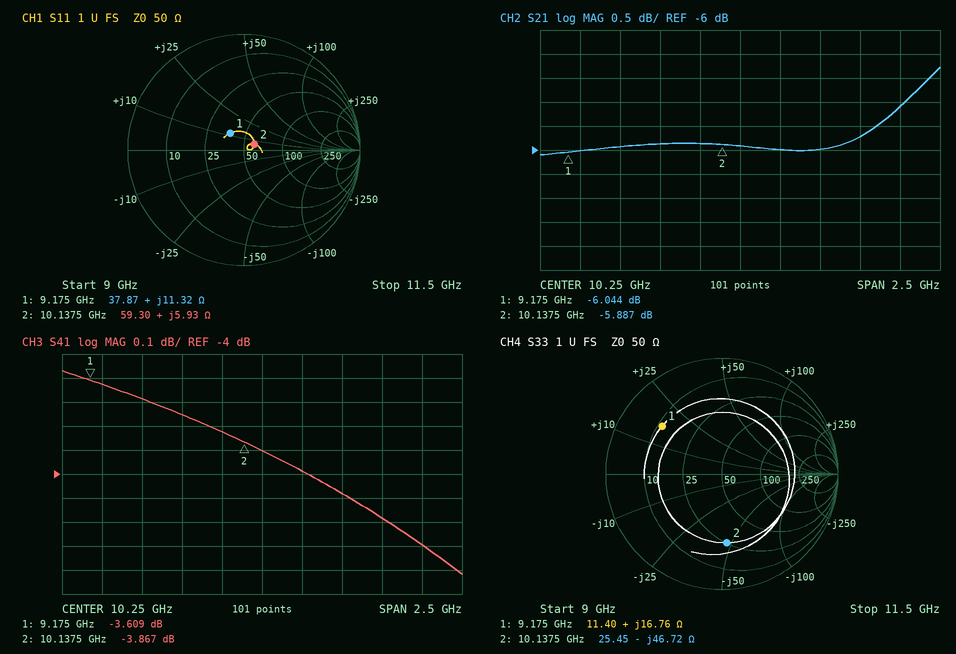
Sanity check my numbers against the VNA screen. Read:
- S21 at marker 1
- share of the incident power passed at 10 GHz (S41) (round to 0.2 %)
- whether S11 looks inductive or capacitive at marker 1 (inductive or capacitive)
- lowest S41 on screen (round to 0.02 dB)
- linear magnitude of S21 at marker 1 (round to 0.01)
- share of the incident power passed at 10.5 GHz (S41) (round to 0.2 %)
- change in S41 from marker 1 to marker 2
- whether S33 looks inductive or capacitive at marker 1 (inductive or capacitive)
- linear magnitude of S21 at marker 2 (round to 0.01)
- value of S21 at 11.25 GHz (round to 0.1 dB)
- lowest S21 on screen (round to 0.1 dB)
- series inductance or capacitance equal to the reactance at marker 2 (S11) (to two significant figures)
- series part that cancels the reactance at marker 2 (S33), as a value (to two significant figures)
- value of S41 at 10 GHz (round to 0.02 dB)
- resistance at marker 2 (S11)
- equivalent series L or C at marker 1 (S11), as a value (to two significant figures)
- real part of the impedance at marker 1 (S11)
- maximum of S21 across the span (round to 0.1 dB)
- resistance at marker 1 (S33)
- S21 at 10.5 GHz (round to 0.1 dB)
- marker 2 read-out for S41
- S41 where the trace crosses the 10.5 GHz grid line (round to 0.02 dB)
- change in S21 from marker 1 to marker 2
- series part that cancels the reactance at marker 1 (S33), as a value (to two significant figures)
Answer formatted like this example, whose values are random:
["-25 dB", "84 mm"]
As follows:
["-6.044 dB", "41.4 %", "inductive", "-4.42 dB", "0.50", "40.0 %", "-0.258 dB", "inductive", "0.51", "-5.1 dB", "-6.1 dB", "93 pH", "730 pH", "-3.82 dB", "59.30 Ω", "200 pH", "37.87 Ω", "-4.3 dB", "11.40 Ω", "-6.0 dB", "-3.867 dB", "-3.98 dB", "0.157 dB", "1.0 pF"]
